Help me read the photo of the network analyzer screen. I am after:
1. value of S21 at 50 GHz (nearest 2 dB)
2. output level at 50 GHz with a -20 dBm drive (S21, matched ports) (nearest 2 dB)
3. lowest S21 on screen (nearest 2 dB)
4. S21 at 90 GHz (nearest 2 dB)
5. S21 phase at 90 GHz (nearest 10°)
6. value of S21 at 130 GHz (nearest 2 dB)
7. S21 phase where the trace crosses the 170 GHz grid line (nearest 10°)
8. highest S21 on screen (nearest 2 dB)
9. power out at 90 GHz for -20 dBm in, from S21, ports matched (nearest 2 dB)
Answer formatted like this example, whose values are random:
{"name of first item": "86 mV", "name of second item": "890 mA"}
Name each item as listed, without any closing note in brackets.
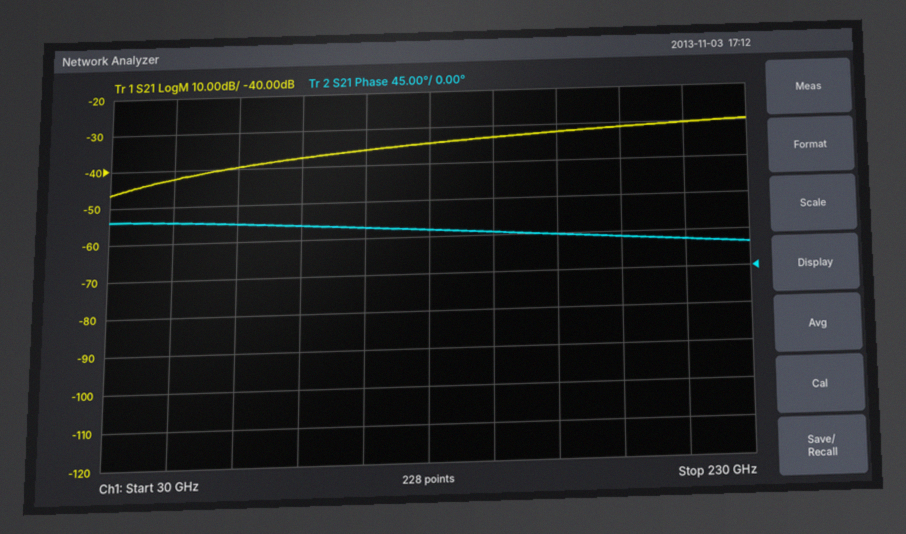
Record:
{"value of S21 at 50 GHz": "-42 dB", "output level at 50 GHz with a -20 dBm drive (S21, matched ports)": "-62 dBm", "lowest S21 on screen": "-46 dB", "S21 at 90 GHz": "-38 dB", "S21 phase at 90 GHz": "60°", "value of S21 at 130 GHz": "-34 dB", "S21 phase where the trace crosses the 170 GHz grid line": "40°", "highest S21 on screen": "-30 dB", "power out at 90 GHz for -20 dBm in, from S21, ports matched": "-58 dBm"}
